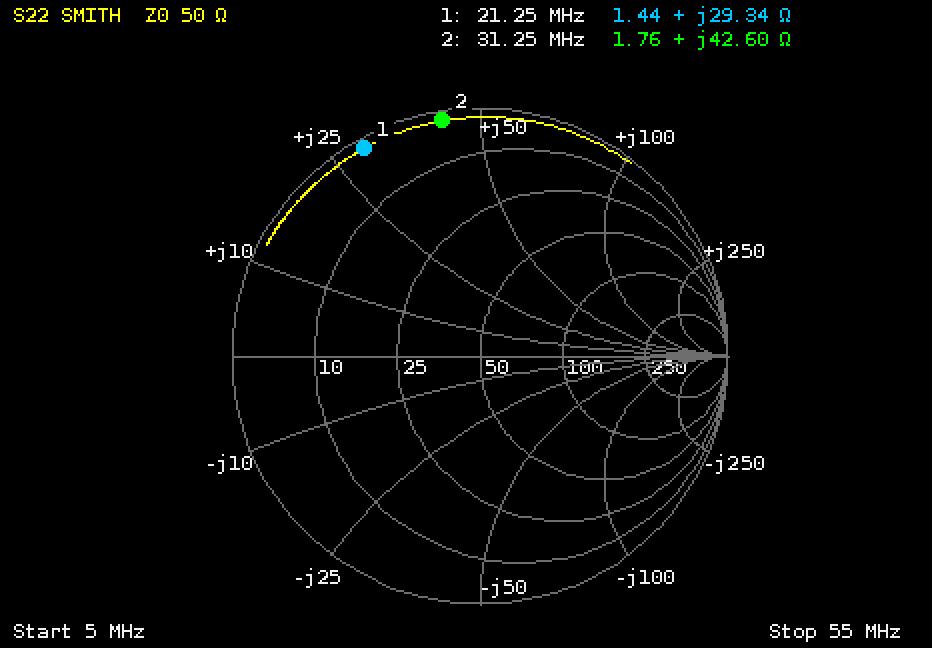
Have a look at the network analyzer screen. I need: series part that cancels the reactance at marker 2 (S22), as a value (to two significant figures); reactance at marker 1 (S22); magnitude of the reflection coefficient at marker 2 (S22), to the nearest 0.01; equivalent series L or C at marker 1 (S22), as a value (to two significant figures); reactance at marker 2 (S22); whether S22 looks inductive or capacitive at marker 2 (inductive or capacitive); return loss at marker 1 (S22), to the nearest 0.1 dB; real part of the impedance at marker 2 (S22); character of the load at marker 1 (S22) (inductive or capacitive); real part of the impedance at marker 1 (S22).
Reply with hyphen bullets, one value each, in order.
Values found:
- 120 pF
- +29.34 Ω
- 0.96
- 220 nH
- +42.60 Ω
- inductive
- 0.4 dB
- 1.76 Ω
- inductive
- 1.44 Ω
